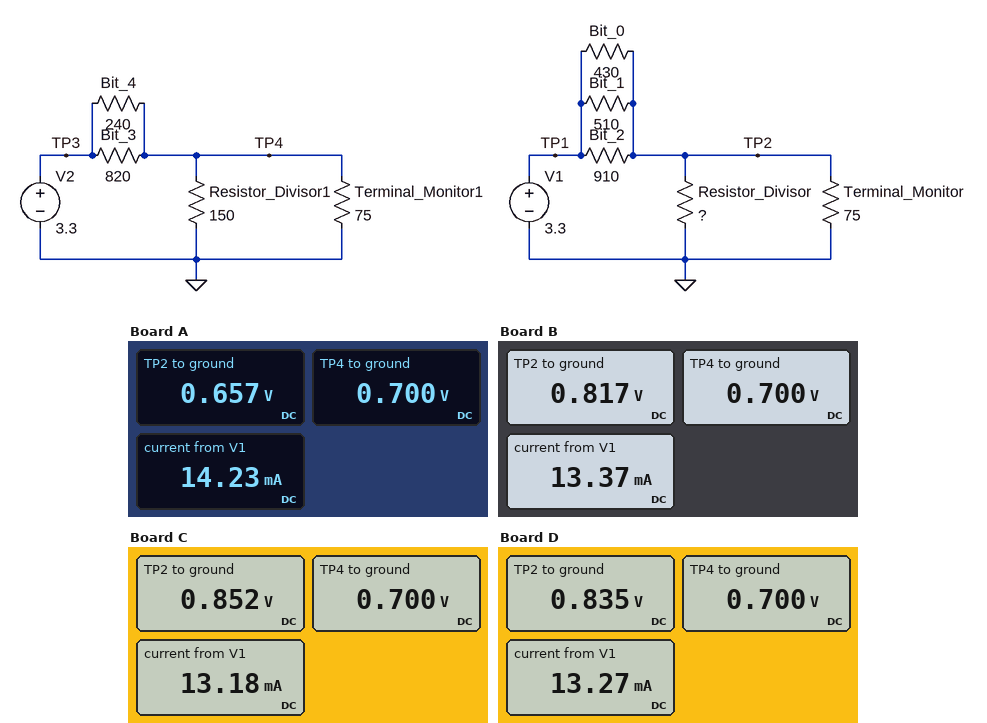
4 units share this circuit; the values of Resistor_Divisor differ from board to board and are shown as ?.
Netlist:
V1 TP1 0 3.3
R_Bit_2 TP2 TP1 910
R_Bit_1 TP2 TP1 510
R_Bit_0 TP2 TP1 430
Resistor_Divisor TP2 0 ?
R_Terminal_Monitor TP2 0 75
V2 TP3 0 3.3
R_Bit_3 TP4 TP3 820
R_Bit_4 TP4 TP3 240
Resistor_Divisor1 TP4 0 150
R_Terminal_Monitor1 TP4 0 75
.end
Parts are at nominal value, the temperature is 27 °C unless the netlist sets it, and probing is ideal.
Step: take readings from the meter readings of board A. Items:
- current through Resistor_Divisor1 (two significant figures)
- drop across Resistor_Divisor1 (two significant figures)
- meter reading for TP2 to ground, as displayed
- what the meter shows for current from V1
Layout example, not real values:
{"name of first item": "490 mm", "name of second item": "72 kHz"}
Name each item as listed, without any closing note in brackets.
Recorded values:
{"current through Resistor_Divisor1": "4.7 mA", "drop across Resistor_Divisor1": "700 mV", "meter reading for TP2 to ground, as displayed": "0.657 V", "what the meter shows for current from V1": "14.23 mA"}
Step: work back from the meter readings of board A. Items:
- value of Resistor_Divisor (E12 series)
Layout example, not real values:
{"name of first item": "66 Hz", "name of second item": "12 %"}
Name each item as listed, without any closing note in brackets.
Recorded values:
{"value of Resistor_Divisor": "120 Ω"}
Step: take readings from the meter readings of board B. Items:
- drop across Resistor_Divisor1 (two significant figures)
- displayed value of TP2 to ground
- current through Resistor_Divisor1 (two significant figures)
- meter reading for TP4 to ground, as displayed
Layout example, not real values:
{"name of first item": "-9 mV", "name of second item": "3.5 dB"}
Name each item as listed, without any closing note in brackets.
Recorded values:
{"drop across Resistor_Divisor1": "700 mV", "displayed value of TP2 to ground": "0.817 V", "current through Resistor_Divisor1": "4.7 mA", "meter reading for TP4 to ground, as displayed": "0.700 V"}
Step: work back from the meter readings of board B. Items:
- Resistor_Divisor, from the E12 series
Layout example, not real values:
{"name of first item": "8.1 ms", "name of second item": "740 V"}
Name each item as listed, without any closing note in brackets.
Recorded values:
{"Resistor_Divisor, from the E12 series": "330 Ω"}
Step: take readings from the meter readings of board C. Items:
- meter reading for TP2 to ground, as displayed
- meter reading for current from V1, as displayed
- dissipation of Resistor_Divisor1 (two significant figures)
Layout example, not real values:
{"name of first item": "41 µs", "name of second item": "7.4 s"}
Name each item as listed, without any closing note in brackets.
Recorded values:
{"meter reading for TP2 to ground, as displayed": "0.852 V", "meter reading for current from V1, as displayed": "13.18 mA", "dissipation of Resistor_Divisor1": "3.3 mW"}
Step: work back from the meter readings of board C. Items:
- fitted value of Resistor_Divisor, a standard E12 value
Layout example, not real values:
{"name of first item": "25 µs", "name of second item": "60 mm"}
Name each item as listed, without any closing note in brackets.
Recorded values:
{"fitted value of Resistor_Divisor, a standard E12 value": "470 Ω"}
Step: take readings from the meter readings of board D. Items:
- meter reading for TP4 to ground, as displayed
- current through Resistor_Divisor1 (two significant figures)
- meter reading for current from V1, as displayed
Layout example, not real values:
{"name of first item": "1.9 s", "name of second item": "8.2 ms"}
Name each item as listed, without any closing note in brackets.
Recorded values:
{"meter reading for TP4 to ground, as displayed": "0.700 V", "current through Resistor_Divisor1": "4.7 mA", "meter reading for current from V1, as displayed": "13.27 mA"}
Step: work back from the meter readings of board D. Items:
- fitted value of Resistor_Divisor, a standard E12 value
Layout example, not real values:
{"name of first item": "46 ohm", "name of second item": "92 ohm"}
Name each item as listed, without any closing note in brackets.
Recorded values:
{"fitted value of Resistor_Divisor, a standard E12 value": "390 Ω"}
